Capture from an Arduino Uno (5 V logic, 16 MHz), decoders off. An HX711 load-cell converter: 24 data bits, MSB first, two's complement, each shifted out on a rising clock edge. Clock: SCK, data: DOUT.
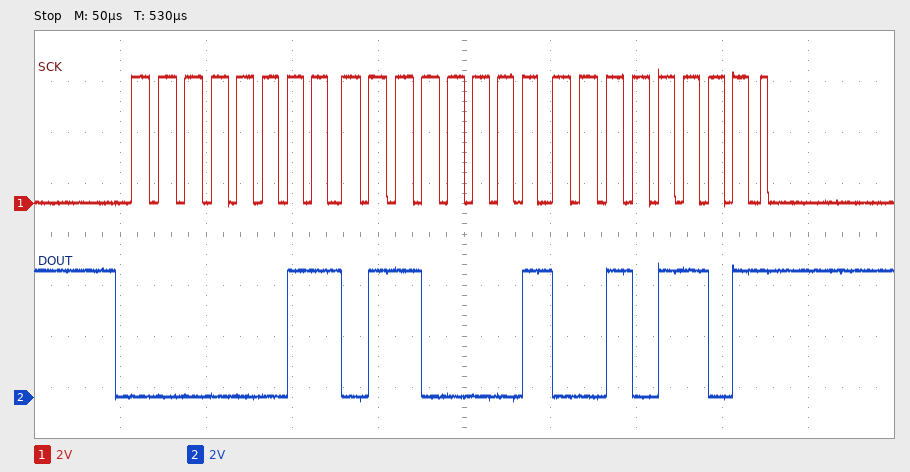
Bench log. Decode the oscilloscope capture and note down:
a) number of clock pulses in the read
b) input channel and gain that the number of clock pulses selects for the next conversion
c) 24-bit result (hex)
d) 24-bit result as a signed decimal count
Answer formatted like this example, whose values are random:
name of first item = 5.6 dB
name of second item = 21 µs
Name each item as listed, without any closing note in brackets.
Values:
number of clock pulses in the read = 25
input channel and gain that the number of clock pulses selects for the next conversion = channel A, gain 128
24-bit result = 0x03612D
24-bit result as a signed decimal count = 221485
